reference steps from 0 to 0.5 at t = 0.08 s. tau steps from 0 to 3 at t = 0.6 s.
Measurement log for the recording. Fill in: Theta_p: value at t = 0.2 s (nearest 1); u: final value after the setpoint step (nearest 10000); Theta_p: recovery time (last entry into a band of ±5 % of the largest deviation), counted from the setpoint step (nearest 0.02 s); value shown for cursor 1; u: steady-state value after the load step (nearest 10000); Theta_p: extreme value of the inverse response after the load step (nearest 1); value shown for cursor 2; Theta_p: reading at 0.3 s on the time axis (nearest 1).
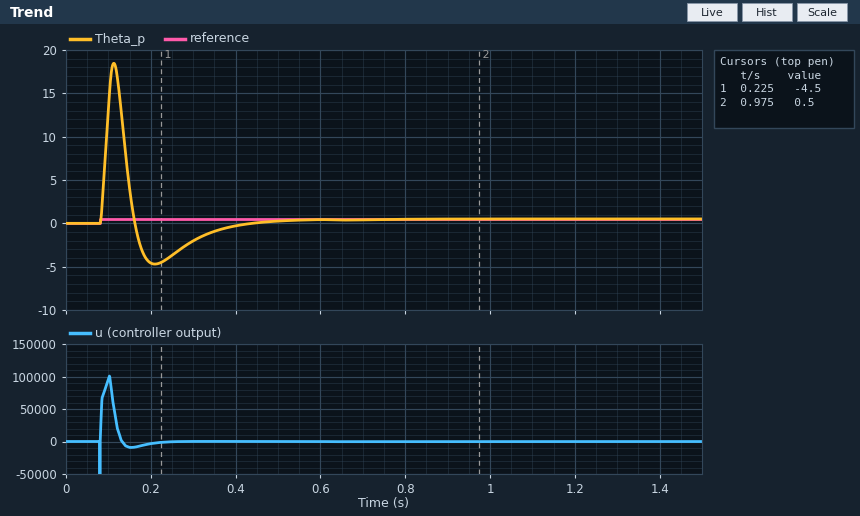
-5
0
0.30 s
-4.5
0
0
0.5
-2
